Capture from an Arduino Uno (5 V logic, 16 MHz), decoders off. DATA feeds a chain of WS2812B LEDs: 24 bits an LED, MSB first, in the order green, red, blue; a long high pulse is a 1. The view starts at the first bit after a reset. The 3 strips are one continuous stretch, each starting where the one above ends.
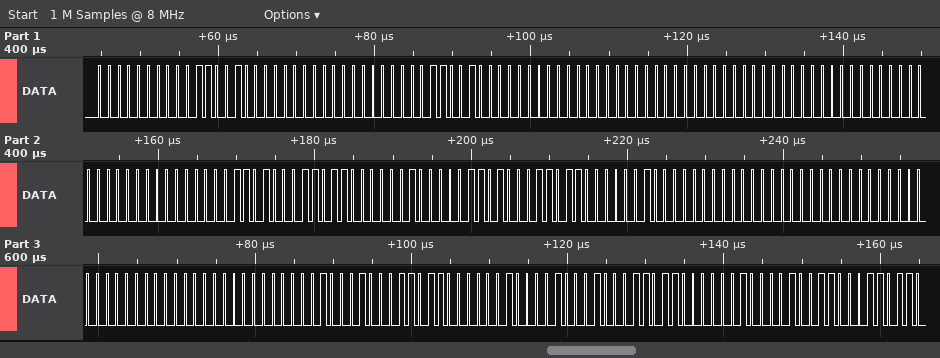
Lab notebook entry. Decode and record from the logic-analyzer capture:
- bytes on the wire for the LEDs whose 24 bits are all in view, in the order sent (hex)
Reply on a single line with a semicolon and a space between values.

00 32 00 00 32 00 00 00 00 00 00 00 0D 1B 02 0D 1B 02 00 00 00 00 00 00 11 1B 02 11 1B 02
